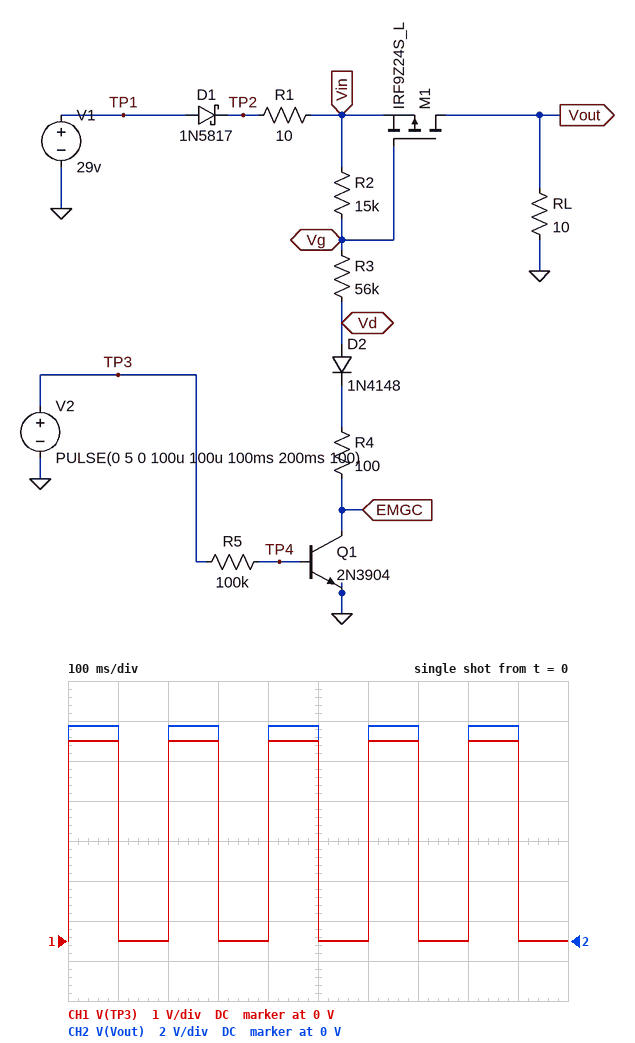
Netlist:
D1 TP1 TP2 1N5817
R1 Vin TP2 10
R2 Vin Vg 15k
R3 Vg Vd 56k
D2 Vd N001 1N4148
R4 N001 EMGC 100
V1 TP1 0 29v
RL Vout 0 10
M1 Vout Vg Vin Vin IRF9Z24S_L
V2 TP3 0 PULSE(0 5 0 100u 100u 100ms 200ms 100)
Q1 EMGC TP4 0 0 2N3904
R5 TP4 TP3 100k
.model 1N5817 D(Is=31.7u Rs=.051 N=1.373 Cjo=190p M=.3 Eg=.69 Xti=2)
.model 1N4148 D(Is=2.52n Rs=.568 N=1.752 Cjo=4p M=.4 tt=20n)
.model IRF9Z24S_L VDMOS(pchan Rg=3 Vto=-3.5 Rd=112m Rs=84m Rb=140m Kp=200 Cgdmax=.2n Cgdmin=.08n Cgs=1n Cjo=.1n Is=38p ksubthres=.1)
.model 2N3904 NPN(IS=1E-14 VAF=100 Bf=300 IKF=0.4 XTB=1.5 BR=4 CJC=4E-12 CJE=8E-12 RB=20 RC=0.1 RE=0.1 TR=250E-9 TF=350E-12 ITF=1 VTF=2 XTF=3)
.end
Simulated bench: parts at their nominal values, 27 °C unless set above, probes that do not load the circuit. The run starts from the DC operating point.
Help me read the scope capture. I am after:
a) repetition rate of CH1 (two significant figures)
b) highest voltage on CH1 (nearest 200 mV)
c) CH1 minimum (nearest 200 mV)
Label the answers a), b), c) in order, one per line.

a) 5.0 Hz
b) 5.0 V
c) 0 V
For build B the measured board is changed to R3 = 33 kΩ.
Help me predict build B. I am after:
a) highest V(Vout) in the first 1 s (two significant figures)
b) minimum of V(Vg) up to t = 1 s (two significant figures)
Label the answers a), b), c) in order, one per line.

a) 14 V
b) 10 V
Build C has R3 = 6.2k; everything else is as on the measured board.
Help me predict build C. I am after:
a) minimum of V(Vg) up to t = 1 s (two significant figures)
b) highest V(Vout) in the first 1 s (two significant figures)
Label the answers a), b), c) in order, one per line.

a) 4.7 V
b) 14 V
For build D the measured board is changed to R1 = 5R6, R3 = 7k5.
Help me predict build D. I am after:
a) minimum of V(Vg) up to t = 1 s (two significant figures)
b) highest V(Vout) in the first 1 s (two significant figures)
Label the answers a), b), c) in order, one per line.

a) 6.6 V
b) 18 V
